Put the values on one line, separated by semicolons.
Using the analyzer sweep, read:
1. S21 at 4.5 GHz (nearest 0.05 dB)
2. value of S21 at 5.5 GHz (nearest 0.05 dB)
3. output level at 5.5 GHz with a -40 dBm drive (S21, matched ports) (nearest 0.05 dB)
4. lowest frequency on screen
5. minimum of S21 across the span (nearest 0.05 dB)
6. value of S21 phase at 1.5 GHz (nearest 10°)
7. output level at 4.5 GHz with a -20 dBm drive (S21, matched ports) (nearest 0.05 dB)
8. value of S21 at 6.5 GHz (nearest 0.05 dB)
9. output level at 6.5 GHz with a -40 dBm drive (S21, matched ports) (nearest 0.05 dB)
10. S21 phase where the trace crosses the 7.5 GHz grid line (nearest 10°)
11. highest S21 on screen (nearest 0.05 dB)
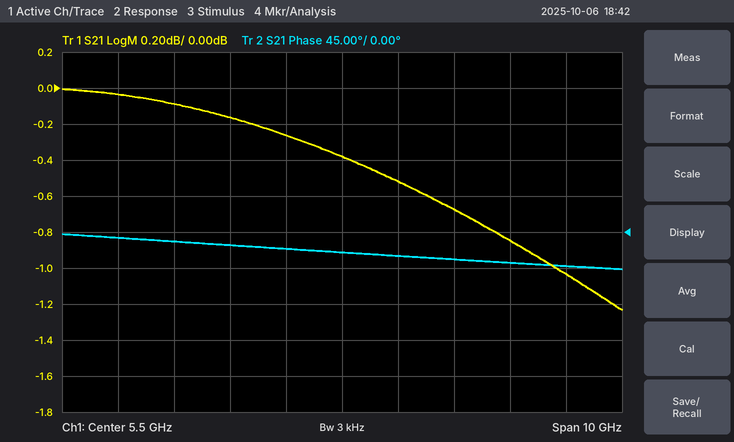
-0.25 dB; -0.40 dB; -40.40 dBm; 500 MHz; -1.25 dB; -10°; -20.25 dBm; -0.50 dB; -40.50 dBm; -30°; 0.00 dB
